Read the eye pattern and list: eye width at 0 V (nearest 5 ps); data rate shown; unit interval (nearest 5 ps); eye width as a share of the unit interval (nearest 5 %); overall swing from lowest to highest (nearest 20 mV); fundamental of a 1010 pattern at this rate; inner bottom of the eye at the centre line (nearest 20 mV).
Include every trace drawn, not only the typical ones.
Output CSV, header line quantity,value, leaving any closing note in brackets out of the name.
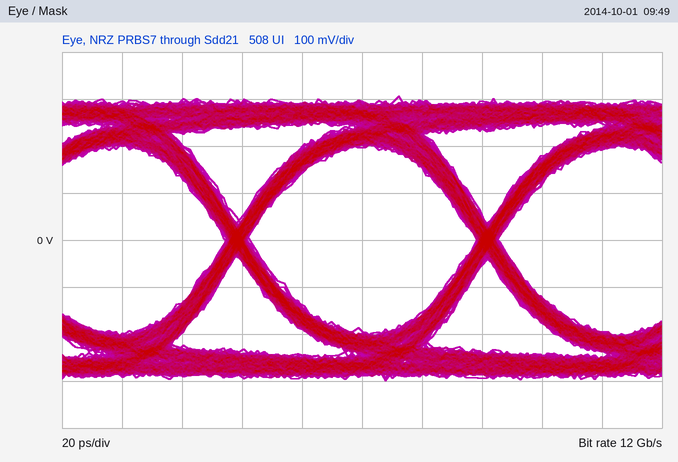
quantity,value
eye width at 0 V,75 ps
data rate shown,12 Gb/s
unit interval,85 ps
eye width as a share of the unit interval,90 %
overall swing from lowest to highest,600 mV
fundamental of a 1010 pattern at this rate,6 GHz
inner bottom of the eye at the centre line,-200 mV
